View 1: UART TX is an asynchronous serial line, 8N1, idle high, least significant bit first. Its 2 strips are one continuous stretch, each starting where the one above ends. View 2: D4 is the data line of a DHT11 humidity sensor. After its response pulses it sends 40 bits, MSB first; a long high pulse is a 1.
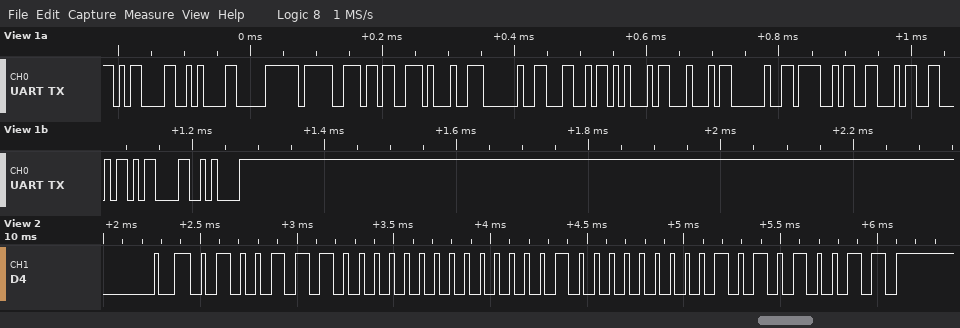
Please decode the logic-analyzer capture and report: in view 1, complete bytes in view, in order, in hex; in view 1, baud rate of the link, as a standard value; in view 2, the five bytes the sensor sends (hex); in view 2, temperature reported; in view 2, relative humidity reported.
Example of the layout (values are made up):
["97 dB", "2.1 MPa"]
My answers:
["0D 0A F0 9F 9B 91 20 4C 45 44 20 4F 46 46 0D 0A", "115200 baud", "4E 00 04 01 53", "4.1 °C", "78 %"]
